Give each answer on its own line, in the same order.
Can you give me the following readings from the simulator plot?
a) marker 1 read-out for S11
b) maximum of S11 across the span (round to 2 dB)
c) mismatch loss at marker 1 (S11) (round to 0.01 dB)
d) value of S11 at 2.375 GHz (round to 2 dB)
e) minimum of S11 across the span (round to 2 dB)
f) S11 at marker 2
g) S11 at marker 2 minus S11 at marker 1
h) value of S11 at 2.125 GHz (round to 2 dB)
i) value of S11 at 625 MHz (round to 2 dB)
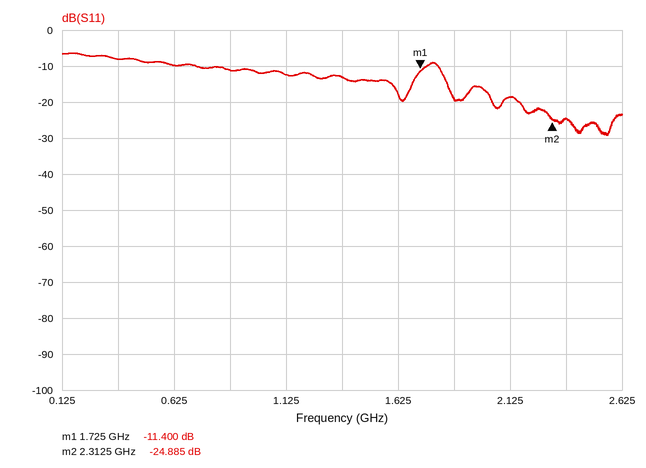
-11.400 dB
-6 dB
0.33 dB
-24 dB
-30 dB
-24.885 dB
-13.485 dB
-18 dB
-10 dB
